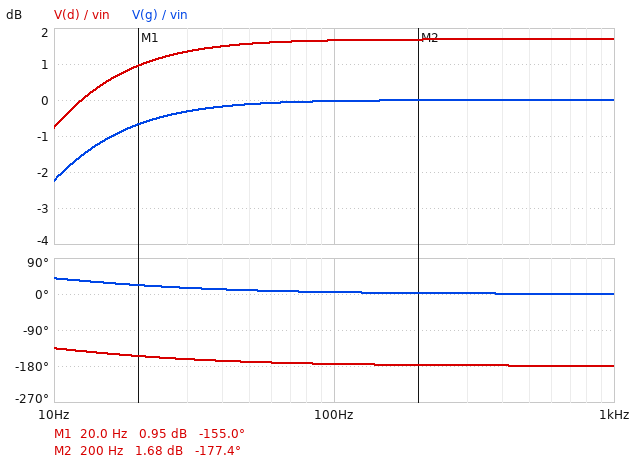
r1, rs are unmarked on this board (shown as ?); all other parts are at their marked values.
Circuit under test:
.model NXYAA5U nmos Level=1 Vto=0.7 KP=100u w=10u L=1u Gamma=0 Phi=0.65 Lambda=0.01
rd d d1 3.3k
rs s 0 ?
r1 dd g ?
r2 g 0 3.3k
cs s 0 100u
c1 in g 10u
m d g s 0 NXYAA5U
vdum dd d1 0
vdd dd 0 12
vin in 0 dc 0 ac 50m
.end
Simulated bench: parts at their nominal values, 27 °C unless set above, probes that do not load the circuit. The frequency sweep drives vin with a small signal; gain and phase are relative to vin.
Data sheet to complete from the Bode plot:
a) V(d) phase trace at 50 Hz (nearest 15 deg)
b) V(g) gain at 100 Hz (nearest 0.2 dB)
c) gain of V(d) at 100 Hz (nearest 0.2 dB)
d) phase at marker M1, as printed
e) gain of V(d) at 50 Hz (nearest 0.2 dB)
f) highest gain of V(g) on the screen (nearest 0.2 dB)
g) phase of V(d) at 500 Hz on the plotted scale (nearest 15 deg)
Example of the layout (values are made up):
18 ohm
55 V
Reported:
-165 deg
0 dB
1.6 dB
-155.0 deg
1.6 dB
0 dB
-180 deg
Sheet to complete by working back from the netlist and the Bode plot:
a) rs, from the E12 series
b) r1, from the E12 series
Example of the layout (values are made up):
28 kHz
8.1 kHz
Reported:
680 Ω
4.7 kΩ
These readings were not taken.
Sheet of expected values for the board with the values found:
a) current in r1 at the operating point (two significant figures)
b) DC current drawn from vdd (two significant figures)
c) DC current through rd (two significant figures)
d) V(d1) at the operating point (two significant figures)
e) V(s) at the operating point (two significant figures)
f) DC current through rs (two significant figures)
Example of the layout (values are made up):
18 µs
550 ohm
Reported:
1.5 mA
4.1 mA
2.6 mA
12 V
1.8 V
2.6 mA
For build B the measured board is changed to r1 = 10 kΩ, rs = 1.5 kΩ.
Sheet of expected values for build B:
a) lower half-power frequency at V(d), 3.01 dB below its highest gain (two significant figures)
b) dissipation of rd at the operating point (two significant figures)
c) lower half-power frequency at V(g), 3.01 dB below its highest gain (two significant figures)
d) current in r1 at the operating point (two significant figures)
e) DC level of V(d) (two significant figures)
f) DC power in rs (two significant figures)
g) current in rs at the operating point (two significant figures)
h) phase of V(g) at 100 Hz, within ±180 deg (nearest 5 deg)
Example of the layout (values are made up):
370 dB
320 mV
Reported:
7.4 Hz
1.8 mW
6.4 Hz
900 µA
9.6 V
820 µW
740 µA
5 deg
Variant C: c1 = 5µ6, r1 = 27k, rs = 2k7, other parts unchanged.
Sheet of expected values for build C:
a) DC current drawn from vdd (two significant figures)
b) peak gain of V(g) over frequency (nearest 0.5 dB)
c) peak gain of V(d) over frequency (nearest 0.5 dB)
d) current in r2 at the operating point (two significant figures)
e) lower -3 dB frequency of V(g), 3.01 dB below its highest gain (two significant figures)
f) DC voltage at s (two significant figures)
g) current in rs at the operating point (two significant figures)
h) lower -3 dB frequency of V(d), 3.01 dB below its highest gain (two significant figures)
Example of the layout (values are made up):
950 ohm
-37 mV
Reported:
480 µA
0 dB
3.0 dB
400 µA
9.7 Hz
220 mV
82 µA
9.8 Hz
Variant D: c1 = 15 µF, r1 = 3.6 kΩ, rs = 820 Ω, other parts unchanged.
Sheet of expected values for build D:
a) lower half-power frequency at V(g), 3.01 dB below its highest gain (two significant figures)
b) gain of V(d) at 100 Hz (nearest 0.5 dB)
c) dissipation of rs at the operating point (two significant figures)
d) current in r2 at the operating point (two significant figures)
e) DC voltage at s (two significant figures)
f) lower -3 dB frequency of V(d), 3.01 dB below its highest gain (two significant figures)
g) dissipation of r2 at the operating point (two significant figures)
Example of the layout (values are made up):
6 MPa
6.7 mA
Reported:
6.2 Hz
-5.5 dB
5.7 mW
1.7 mA
2.2 V
6.6 Hz
10 mW
